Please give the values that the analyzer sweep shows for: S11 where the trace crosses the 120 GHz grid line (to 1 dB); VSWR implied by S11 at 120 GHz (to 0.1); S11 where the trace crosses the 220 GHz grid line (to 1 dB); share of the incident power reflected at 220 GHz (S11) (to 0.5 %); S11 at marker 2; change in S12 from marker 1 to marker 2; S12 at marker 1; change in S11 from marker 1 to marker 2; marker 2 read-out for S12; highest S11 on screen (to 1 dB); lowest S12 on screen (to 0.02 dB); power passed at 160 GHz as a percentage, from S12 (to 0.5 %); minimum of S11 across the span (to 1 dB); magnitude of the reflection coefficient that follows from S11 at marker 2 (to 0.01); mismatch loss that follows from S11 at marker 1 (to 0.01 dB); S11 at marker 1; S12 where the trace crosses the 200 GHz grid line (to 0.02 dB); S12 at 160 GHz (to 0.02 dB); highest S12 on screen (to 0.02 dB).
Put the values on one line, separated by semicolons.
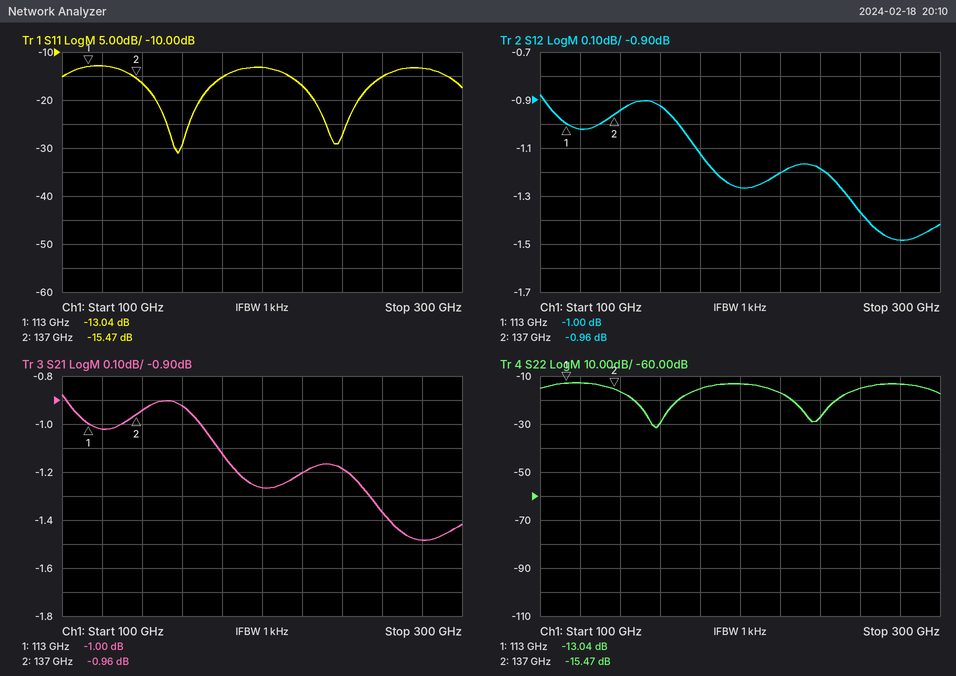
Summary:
-13 dB; 1.6; -17 dB; 2.0 %; -15.47 dB; 0.04 dB; -1.00 dB; -2.43 dB; -0.96 dB; -13 dB; -1.48 dB; 81.0 %; -31 dB; 0.17; 0.22 dB; -13.04 dB; -1.26 dB; -0.92 dB; -0.88 dB
